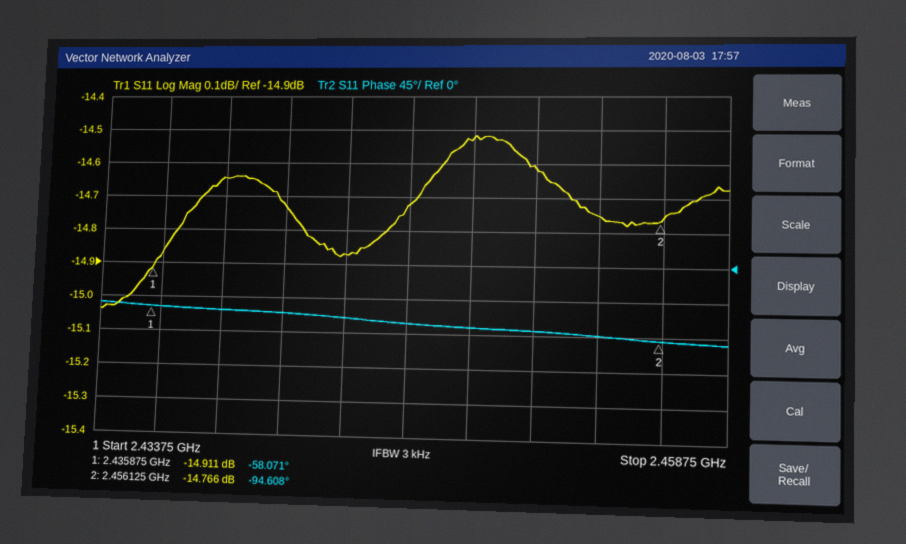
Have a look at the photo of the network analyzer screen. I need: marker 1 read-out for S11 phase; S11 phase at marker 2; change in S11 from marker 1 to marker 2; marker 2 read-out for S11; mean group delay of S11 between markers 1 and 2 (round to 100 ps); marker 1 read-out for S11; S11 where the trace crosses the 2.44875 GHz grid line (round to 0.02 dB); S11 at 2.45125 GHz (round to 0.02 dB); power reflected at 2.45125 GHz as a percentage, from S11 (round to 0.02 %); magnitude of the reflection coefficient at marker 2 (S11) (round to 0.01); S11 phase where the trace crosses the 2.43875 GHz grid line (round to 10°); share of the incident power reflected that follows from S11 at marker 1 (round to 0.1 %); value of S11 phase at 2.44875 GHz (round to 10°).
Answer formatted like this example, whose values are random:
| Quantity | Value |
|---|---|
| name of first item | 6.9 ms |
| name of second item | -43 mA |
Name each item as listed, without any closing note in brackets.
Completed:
| Quantity | Value |
|---|---|
| marker 1 read-out for S11 phase | -58.071° |
| S11 phase at marker 2 | -94.608° |
| change in S11 from marker 1 to marker 2 | 0.145 dB |
| marker 2 read-out for S11 | -14.766 dB |
| mean group delay of S11 between markers 1 and 2 | 5.0 ns |
| marker 1 read-out for S11 | -14.911 dB |
| S11 where the trace crosses the 2.44875 GHz grid line | -14.52 dB |
| S11 at 2.45125 GHz | -14.62 dB |
| power reflected at 2.45125 GHz as a percentage, from S11 | 3.46 % |
| magnitude of the reflection coefficient at marker 2 (S11) | 0.18 |
| S11 phase where the trace crosses the 2.43875 GHz grid line | -60° |
| share of the incident power reflected that follows from S11 at marker 1 | 3.2 % |
| value of S11 phase at 2.44875 GHz | -80° |
